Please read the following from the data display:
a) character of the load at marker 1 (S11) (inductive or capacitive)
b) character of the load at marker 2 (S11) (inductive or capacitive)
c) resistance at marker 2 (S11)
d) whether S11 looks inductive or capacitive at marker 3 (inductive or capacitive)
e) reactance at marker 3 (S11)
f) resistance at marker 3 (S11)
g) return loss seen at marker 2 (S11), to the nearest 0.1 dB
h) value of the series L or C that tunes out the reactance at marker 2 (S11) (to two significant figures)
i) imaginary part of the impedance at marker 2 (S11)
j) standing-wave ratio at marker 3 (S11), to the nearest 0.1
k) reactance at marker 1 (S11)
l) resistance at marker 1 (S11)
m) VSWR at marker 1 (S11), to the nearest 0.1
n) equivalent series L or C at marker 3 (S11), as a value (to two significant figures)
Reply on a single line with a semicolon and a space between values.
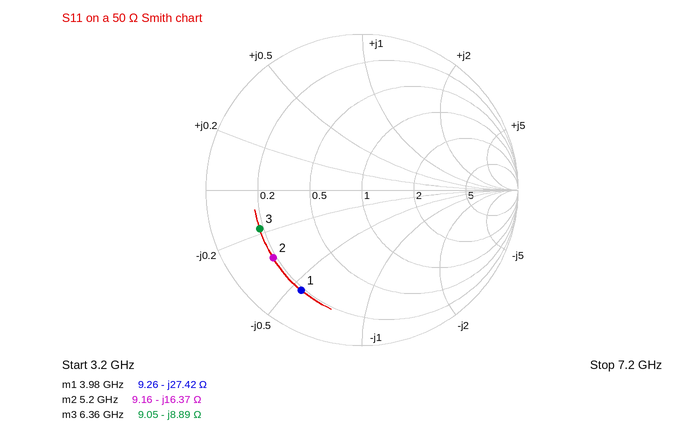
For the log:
capacitive; capacitive; 9.16 Ω; capacitive; -8.89 Ω; 9.05 Ω; 2.9 dB; 500 pH; -16.37 Ω; 5.7; -27.42 Ω; 9.26 Ω; 7.1; 2.8 pF
